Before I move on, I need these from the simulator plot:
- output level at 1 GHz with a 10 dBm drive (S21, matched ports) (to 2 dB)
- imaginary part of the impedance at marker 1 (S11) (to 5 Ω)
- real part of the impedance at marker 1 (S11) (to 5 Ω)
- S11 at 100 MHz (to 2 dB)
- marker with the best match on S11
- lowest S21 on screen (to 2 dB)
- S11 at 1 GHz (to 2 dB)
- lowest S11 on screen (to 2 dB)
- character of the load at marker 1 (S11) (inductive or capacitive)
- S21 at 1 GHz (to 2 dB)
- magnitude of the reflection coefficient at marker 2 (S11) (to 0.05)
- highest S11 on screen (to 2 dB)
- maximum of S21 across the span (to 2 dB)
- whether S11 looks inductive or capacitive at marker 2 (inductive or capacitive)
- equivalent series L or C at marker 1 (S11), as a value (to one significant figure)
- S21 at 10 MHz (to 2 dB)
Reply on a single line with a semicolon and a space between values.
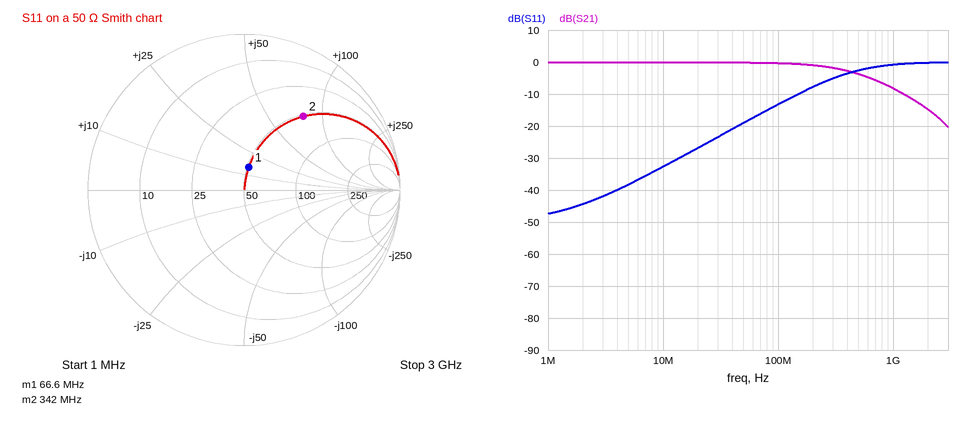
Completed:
2 dBm; +15 Ω; 50 Ω; -14 dB; marker 1; -20 dB; 0 dB; -48 dB; inductive; -8 dB; 0.60; 0 dB; 0 dB; inductive; 40 nH; 0 dB
